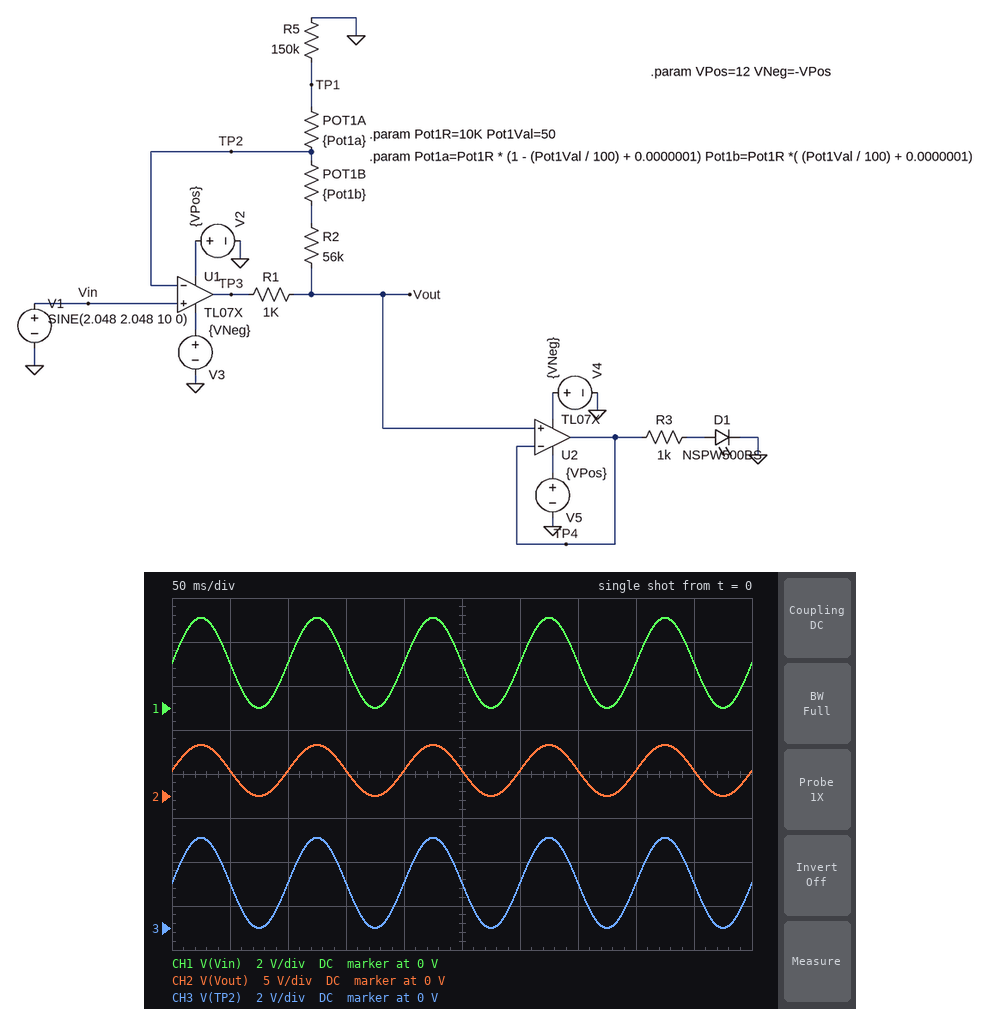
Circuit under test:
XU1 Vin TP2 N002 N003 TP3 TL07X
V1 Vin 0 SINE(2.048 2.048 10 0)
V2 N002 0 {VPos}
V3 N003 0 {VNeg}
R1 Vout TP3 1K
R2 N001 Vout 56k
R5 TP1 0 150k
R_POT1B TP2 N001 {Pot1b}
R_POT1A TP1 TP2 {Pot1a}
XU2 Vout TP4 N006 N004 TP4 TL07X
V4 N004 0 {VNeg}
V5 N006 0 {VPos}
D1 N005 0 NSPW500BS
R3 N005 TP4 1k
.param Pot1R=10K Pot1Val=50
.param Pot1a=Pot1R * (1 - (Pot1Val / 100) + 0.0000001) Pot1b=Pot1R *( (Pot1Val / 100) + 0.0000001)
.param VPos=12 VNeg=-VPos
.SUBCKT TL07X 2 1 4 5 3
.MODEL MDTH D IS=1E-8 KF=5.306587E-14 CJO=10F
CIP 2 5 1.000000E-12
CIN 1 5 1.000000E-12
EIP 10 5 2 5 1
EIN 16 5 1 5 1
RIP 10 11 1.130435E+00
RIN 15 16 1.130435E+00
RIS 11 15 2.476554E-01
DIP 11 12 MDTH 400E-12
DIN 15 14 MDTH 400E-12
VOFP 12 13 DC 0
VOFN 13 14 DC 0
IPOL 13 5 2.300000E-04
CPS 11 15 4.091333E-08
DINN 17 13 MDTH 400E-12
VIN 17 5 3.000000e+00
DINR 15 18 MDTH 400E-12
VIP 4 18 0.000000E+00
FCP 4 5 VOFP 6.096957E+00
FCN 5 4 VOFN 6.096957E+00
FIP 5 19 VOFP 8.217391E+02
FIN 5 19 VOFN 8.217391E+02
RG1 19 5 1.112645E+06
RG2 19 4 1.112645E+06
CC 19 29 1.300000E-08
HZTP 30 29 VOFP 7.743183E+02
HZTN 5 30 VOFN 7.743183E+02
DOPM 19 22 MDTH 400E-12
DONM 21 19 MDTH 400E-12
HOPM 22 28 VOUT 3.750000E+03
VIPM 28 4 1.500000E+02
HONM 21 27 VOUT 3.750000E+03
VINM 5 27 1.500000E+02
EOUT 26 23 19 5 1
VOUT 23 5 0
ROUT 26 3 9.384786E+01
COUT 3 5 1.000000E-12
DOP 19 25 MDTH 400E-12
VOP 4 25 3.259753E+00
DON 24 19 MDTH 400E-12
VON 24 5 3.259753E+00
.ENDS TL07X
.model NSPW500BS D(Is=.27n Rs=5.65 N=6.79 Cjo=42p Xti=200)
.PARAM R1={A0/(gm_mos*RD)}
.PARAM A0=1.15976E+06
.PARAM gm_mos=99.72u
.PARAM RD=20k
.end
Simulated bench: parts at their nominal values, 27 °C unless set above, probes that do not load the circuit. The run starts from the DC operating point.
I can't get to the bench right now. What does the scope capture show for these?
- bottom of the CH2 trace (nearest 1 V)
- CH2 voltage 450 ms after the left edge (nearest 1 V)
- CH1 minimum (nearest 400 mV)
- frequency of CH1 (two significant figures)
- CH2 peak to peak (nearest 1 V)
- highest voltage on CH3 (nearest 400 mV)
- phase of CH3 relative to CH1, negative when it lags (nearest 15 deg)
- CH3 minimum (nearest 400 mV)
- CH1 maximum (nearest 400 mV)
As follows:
0 V
3 V
0 V
10 Hz
6 V
4.0 V
0 deg
0 V
4.0 V
